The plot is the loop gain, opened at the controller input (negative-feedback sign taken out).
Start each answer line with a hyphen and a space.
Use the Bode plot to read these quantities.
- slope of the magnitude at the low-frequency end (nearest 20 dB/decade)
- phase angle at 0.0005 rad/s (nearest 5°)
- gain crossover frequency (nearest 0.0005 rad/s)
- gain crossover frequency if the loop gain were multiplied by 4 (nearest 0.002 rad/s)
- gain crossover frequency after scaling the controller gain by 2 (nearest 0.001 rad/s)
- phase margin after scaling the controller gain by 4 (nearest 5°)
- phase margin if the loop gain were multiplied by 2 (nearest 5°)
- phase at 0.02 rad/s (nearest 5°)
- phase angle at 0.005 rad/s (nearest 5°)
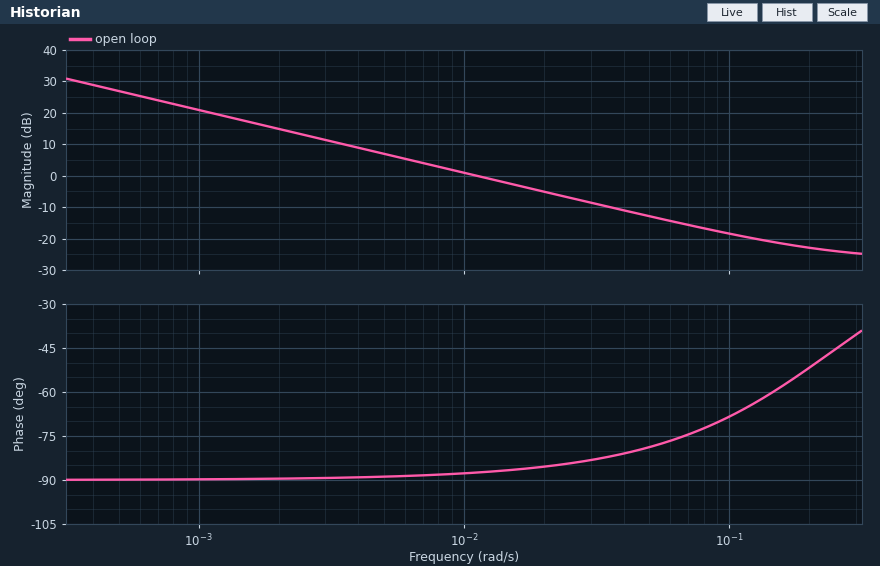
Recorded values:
- -20 dB/decade
- -90°
- 0.0110 rad/s
- 0.046 rad/s
- 0.022 rad/s
- 100°
- 95°
- -85°
- -90°
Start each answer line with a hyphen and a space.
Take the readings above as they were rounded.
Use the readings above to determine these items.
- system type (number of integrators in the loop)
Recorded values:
- 1
